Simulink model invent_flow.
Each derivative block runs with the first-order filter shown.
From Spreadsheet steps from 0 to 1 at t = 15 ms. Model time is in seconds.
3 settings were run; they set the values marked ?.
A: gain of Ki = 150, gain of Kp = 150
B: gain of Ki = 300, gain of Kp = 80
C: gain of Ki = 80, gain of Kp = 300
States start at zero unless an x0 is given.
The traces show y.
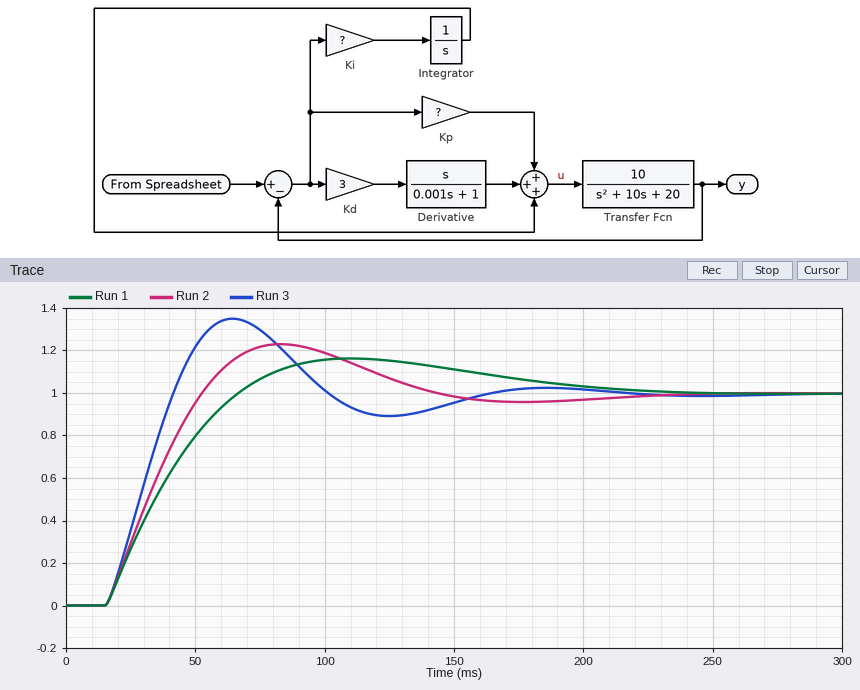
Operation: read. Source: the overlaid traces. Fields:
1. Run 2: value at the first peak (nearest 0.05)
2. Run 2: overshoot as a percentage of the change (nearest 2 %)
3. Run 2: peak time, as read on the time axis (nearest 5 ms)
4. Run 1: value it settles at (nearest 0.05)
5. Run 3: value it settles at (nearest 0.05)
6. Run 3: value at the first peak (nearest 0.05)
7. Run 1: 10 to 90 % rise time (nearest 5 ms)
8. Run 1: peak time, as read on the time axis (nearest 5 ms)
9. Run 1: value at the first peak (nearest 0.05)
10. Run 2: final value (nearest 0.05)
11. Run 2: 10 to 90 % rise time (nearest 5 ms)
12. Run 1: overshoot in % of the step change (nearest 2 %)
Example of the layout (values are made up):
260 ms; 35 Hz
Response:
1.25; 24 %; 85 ms; 1.00; 1.00; 1.35; 40 ms; 110 ms; 1.15; 1.00; 30 ms; 16 %
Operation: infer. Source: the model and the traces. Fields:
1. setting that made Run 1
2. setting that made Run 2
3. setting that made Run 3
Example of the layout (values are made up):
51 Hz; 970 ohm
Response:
B; A; C
